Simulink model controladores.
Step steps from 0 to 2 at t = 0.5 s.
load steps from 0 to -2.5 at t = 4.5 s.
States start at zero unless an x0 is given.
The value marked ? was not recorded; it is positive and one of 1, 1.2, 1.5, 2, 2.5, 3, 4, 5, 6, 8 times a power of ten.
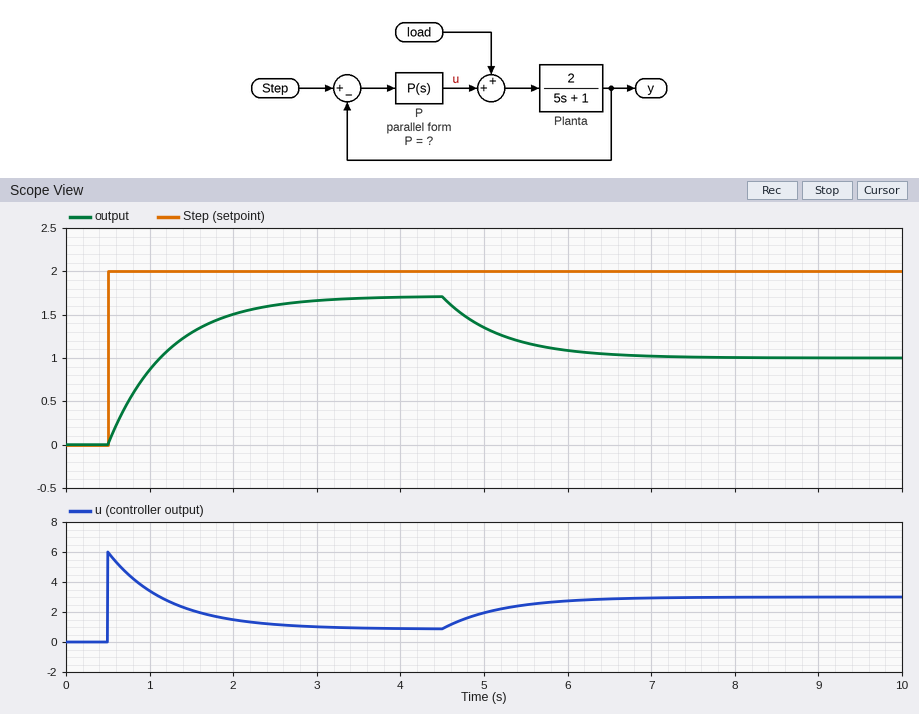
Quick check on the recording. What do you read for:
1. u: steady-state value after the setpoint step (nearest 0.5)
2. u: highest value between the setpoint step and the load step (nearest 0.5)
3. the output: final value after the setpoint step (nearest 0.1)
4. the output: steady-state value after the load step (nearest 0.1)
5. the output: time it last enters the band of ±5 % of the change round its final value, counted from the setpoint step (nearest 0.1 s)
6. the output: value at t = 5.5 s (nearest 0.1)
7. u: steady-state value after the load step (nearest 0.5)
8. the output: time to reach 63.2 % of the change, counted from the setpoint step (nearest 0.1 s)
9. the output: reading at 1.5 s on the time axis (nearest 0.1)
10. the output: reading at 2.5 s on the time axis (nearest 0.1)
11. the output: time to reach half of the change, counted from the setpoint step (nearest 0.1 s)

1.0
6.0
1.7
1.0
2.1 s
1.2
3.0
0.7 s
1.3
1.6
0.5 s
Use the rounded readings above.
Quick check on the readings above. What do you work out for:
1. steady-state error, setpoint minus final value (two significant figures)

0.30
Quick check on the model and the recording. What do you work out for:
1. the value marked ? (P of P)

3
